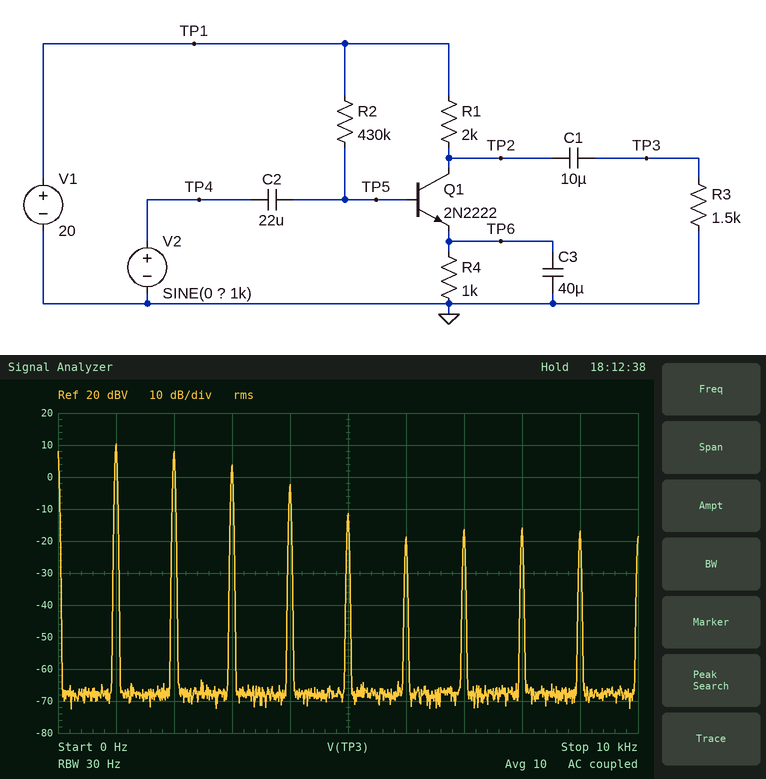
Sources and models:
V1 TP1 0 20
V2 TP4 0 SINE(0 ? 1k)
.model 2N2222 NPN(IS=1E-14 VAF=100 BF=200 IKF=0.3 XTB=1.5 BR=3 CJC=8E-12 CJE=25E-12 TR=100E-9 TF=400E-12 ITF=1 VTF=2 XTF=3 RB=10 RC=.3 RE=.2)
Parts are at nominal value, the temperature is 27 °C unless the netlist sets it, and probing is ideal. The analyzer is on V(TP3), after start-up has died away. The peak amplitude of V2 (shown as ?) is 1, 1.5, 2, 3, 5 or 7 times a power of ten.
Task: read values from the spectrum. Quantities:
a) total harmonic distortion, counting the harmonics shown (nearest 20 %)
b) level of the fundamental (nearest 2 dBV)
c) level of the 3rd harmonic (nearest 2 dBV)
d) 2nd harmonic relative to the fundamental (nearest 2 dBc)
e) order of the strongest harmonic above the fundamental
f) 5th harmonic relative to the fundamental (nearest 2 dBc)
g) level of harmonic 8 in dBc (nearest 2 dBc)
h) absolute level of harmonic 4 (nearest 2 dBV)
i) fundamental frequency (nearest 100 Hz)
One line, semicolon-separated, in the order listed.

100 %; 10 dBV; 4 dBV; -2 dBc; 2; -22 dBc; -26 dBc; -2 dBV; 1.0 kHz
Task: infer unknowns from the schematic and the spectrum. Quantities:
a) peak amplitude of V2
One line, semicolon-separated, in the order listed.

200 mV
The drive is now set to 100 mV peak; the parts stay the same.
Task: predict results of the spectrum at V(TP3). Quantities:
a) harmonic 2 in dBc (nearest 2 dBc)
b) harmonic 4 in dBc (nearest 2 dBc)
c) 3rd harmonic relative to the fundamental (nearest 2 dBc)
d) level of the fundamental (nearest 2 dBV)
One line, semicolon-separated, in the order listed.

-6 dBc; -26 dBc; -14 dBc; 12 dBV
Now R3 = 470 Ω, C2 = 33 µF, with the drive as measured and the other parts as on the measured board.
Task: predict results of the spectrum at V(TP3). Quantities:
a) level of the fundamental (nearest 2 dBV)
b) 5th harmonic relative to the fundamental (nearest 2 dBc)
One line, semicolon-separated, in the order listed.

6 dBV; -20 dBc
